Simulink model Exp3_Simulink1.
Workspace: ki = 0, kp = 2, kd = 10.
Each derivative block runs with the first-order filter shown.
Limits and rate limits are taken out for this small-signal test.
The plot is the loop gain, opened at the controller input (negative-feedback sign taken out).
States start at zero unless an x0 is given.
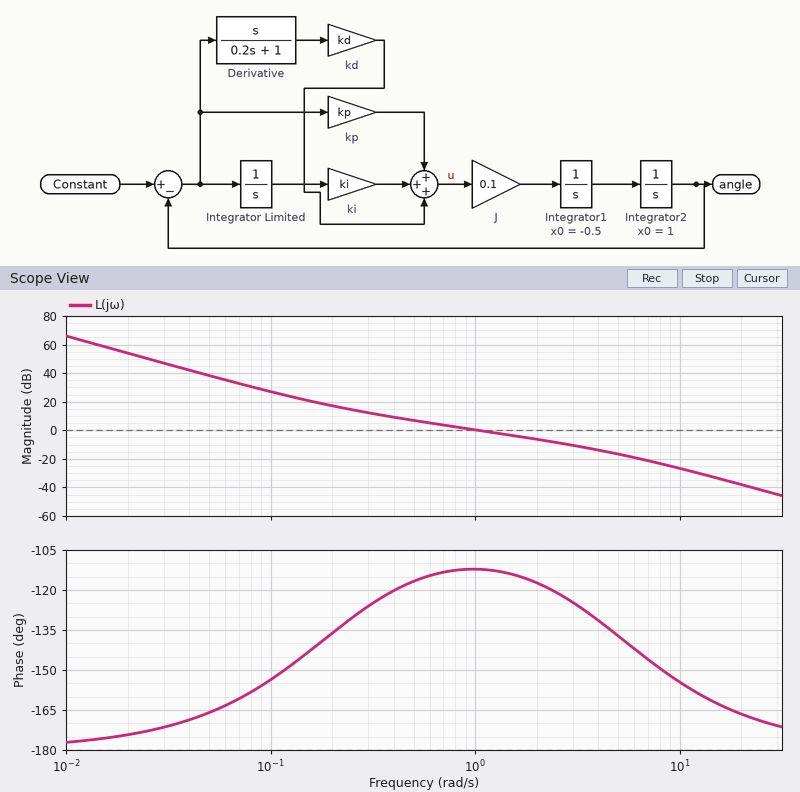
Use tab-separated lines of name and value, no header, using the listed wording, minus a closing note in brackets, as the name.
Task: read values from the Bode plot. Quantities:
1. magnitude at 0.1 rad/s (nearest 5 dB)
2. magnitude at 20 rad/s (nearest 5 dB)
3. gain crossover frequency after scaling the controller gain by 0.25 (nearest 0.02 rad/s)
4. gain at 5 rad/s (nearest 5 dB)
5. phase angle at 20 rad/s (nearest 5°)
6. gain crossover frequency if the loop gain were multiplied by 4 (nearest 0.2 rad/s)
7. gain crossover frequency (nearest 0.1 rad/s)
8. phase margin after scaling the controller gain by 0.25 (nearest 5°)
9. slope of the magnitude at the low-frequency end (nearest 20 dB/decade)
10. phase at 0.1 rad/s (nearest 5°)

magnitude at 0.1 rad/s	25 dB
magnitude at 20 rad/s	-40 dB
gain crossover frequency after scaling the controller gain by 0.25	0.30 rad/s
gain at 5 rad/s	-15 dB
phase angle at 20 rad/s	-165°
gain crossover frequency if the loop gain were multiplied by 4	3.4 rad/s
gain crossover frequency	1.0 rad/s
phase margin after scaling the controller gain by 0.25	55°
slope of the magnitude at the low-frequency end	-40 dB/decade
phase at 0.1 rad/s	-155°
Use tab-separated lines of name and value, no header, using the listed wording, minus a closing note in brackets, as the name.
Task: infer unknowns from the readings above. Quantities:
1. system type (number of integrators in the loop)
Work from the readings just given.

system type	2
